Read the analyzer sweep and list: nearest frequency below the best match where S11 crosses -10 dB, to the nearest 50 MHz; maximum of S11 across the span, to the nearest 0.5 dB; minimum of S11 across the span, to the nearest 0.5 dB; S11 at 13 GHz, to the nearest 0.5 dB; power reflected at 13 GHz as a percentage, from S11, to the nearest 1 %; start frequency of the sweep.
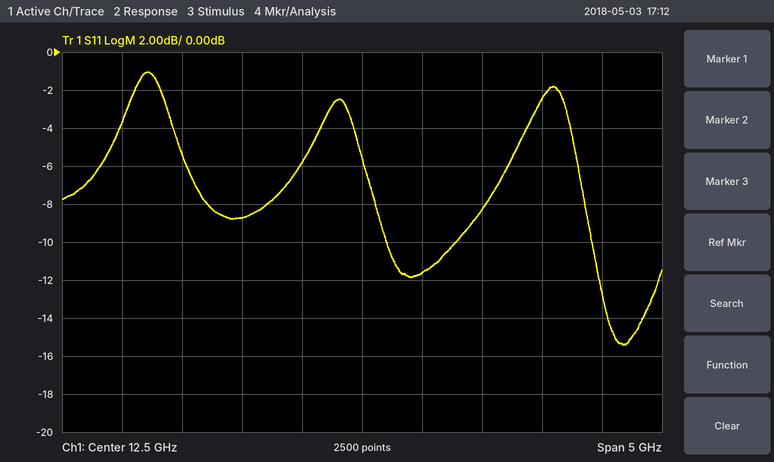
14.40 GHz
-1.0 dB
-15.5 dB
-11.5 dB
7 %
10 GHz
